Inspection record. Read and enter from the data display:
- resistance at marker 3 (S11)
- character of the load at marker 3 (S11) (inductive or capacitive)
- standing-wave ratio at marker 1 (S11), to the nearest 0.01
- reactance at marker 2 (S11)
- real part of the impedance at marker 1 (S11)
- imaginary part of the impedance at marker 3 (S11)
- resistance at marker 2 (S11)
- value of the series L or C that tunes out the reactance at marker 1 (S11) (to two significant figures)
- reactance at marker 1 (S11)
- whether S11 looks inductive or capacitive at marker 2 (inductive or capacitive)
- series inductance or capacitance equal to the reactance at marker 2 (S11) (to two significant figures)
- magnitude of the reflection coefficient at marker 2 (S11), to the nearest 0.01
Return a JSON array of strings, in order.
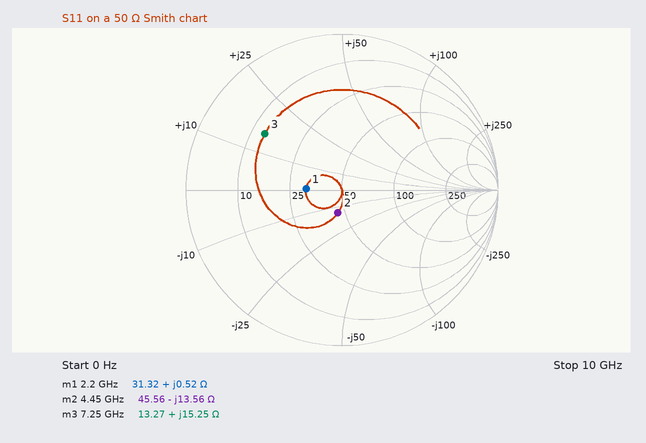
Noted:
["13.27 Ω", "inductive", "1.60", "-13.56 Ω", "31.32 Ω", "+15.25 Ω", "45.56 Ω", "140 pF", "+0.52 Ω", "capacitive", "2.6 pF", "0.15"]
